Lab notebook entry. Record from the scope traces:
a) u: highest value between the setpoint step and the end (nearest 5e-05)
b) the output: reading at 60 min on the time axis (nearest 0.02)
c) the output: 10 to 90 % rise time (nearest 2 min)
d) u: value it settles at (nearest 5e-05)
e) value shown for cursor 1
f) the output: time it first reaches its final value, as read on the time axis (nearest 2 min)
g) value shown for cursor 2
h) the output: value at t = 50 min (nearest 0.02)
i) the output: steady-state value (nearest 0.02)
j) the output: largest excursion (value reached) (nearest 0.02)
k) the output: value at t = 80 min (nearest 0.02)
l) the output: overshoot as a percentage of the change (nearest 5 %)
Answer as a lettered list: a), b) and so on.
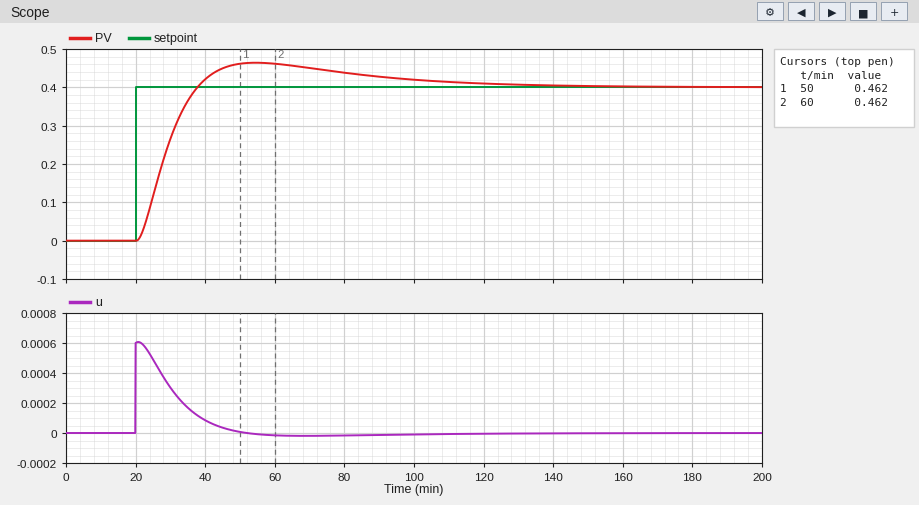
a) 0.00060
b) 0.46
c) 12 min
d) 0.00000
e) 0.462
f) 38 min
g) 0.462
h) 0.46
i) 0.40
j) 0.46
k) 0.44
l) 15 %
